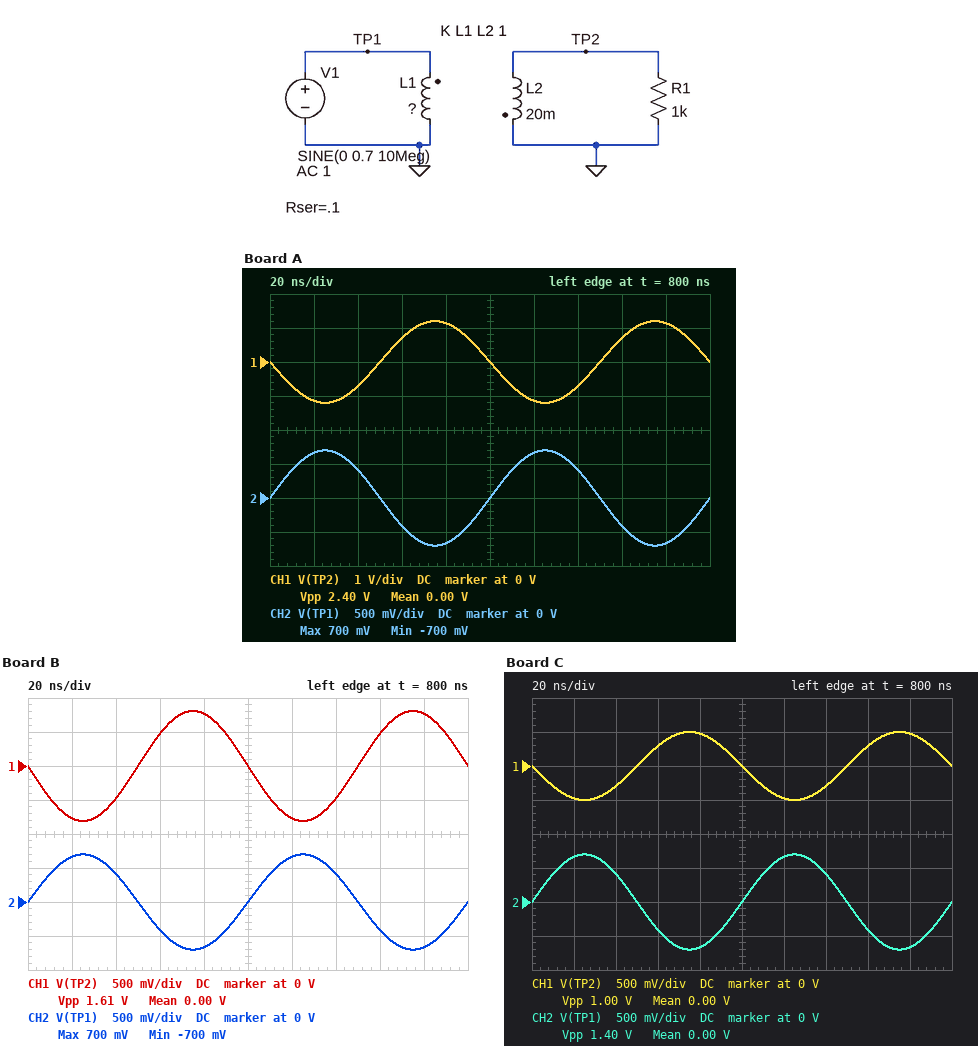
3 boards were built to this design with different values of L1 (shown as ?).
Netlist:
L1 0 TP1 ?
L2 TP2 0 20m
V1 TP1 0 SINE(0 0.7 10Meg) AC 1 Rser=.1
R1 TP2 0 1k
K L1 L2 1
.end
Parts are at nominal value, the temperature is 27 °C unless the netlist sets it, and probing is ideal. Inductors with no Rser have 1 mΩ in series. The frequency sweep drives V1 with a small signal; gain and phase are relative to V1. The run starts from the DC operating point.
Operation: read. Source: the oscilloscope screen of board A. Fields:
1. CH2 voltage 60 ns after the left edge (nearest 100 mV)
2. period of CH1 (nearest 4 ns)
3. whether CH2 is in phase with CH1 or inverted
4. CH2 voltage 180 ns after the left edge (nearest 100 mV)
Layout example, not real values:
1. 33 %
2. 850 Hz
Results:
1. -400 mV
2. 100 ns
3. inverted
4. -700 mV
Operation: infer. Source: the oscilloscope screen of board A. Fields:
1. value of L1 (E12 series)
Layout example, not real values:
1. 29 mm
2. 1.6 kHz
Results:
1. 6.8 mH
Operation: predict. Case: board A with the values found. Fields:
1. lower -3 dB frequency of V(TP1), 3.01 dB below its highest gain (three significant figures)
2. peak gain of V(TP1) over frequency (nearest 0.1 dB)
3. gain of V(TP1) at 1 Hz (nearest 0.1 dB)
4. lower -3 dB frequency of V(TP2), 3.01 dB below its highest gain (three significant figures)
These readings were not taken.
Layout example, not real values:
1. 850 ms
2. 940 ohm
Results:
1. 2.36 Hz
2. 0 dB
3. -8.2 dB
4. 2.36 Hz
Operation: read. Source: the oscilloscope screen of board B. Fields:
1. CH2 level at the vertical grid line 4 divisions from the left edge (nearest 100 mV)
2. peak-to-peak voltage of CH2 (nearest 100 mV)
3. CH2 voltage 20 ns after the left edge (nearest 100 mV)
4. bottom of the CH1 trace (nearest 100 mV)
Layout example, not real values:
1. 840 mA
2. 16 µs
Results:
1. -700 mV
2. 1.4 V
3. 700 mV
4. -800 mV
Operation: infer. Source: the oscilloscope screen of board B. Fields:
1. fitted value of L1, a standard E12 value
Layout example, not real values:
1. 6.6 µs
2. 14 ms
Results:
1. 15 mH
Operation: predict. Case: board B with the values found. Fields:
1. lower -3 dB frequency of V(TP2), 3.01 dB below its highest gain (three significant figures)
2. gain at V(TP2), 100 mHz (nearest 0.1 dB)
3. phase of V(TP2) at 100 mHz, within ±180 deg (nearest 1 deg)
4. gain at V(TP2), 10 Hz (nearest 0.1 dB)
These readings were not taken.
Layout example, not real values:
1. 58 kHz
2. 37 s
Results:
1. 1.07 Hz
2. -19.4 dB
3. -95 deg
4. 1.2 dB
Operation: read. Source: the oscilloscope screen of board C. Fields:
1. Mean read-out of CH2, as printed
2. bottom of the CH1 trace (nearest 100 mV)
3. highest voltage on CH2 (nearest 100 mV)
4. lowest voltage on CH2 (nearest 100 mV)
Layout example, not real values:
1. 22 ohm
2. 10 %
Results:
1. 0.00 V
2. -500 mV
3. 700 mV
4. -700 mV
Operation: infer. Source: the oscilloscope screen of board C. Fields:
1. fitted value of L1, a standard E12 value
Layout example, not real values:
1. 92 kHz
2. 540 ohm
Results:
1. 39 mH
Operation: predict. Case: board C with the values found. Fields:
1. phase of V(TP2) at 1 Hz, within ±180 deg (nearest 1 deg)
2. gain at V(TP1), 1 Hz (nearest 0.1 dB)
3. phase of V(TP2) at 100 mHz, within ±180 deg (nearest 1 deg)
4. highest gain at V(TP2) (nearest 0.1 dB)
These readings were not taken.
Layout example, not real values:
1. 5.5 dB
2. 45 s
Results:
1. -158 deg
2. -0.7 dB
3. -104 deg
4. -2.9 dB
